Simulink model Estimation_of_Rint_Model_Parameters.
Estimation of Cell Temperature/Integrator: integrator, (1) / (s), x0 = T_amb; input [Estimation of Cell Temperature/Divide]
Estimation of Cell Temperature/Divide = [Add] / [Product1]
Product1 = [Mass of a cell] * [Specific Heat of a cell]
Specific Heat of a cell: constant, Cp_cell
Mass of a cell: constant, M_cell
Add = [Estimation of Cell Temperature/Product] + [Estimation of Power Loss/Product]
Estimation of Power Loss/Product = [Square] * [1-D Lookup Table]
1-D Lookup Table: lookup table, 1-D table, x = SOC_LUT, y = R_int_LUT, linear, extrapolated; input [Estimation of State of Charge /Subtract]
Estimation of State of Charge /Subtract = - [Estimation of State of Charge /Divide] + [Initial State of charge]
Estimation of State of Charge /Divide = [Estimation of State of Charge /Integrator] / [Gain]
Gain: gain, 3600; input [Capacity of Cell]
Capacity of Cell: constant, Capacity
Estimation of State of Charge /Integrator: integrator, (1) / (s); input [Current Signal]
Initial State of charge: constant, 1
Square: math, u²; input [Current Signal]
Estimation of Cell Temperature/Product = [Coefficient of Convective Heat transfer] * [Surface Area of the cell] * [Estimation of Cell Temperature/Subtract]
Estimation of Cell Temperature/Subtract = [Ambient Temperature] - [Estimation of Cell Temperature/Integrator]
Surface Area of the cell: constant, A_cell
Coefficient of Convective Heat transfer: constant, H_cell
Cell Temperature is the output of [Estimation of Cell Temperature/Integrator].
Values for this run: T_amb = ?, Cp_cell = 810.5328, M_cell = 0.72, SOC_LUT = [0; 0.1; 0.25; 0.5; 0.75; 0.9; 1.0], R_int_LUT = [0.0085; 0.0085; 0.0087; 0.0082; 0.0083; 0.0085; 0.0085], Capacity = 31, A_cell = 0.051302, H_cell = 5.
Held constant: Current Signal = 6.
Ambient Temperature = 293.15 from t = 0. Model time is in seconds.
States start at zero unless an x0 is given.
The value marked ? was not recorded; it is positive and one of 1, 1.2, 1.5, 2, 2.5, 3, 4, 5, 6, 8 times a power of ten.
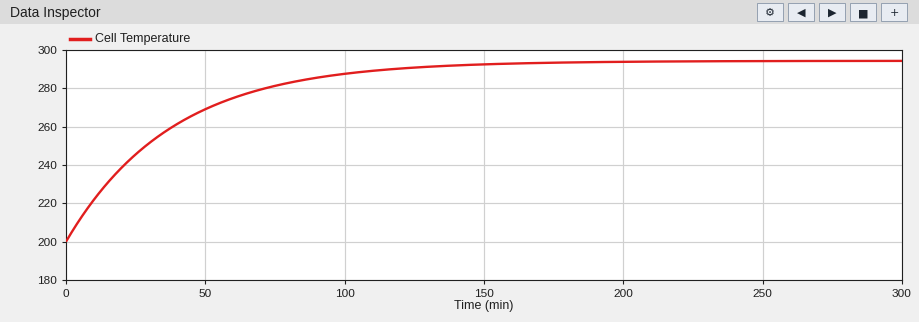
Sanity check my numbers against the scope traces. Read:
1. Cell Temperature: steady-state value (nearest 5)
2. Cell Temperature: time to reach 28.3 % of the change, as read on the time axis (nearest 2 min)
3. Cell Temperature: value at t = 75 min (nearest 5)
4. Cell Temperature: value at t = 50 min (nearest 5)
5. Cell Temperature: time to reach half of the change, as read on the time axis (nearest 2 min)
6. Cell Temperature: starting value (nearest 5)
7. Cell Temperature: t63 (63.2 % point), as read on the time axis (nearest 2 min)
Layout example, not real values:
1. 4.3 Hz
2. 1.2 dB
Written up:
1. 295
2. 12 min
3. 280
4. 270
5. 26 min
6. 200
7. 38 min
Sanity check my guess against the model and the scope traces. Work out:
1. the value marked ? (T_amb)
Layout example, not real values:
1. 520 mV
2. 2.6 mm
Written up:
1. 200
